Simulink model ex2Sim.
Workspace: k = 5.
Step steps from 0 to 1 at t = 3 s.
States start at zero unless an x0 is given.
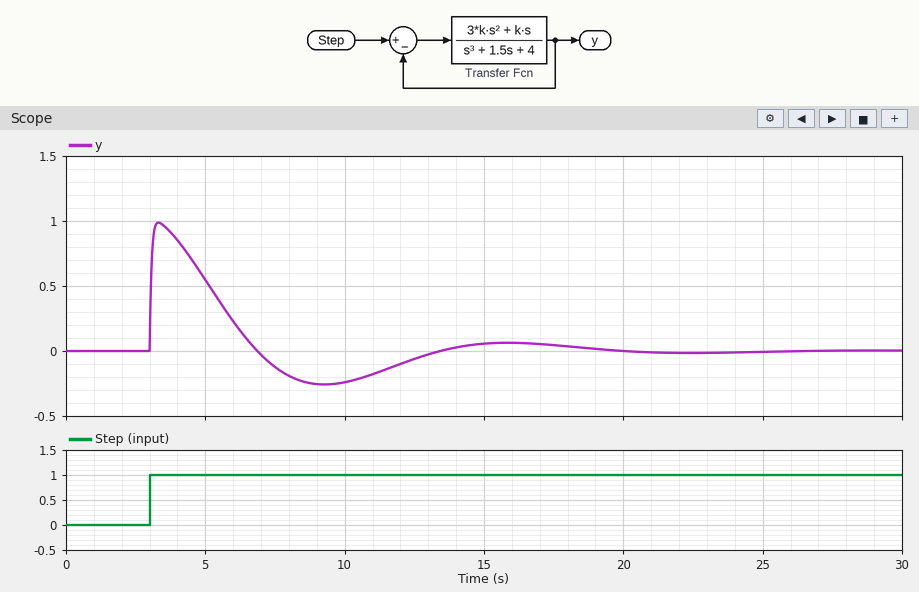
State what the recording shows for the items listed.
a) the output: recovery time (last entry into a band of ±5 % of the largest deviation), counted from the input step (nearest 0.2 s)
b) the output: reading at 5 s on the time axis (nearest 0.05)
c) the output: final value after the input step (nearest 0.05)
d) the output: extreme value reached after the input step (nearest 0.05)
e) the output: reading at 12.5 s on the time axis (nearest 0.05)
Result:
14.2 s
0.55
0.00
1.00
-0.05
